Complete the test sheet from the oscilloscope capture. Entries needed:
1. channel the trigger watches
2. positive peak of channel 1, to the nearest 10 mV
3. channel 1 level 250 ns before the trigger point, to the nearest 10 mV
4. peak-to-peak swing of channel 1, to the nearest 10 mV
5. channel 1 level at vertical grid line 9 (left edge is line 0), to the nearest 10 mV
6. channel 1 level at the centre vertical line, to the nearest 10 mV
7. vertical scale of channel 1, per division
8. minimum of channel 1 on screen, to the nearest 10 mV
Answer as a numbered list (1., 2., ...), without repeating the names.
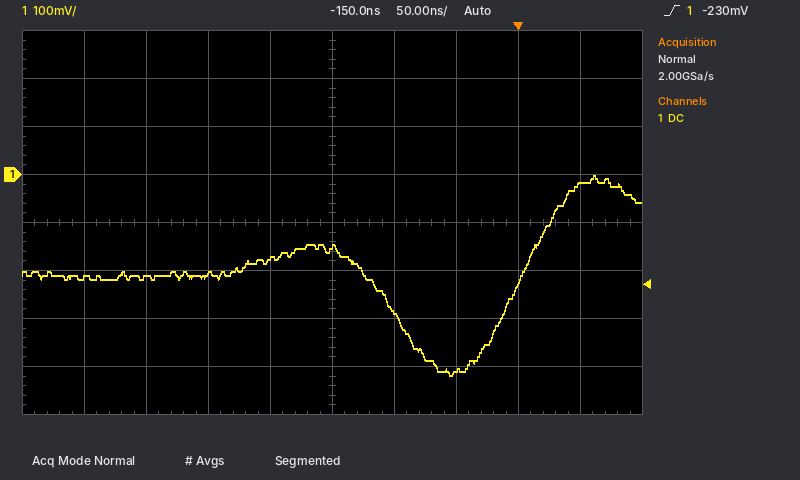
1. channel 1
2. 0 mV
3. -210 mV
4. 420 mV
5. -20 mV
6. -150 mV
7. 100 mV
8. -420 mV
